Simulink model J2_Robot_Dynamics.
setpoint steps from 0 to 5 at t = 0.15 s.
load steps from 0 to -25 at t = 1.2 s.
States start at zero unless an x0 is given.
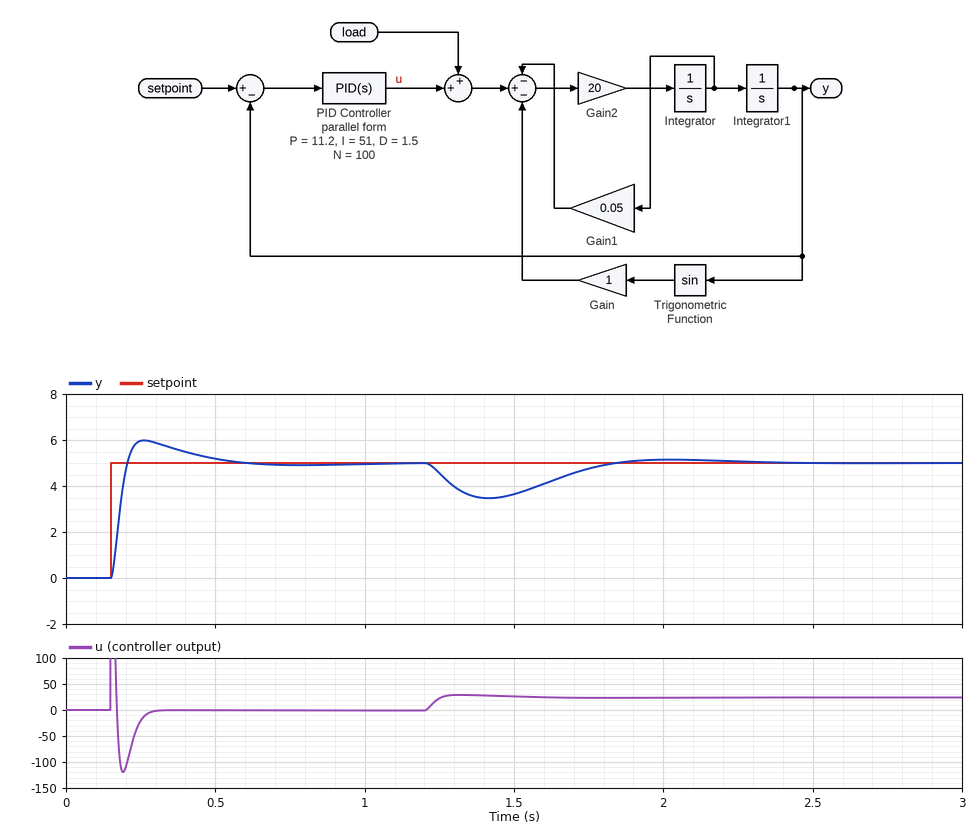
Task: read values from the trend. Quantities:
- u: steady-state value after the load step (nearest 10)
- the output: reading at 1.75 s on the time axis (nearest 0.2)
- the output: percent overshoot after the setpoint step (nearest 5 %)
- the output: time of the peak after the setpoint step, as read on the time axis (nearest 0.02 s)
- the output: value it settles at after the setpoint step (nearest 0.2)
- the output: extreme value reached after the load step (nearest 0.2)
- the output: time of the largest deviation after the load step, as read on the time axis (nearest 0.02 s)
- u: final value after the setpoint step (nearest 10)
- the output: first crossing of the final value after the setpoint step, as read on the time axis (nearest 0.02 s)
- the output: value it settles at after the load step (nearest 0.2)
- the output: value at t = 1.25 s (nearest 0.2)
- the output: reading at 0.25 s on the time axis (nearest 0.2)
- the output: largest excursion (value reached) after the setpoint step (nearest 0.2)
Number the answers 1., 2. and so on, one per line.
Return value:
1. 20
2. 4.8
3. 20 %
4. 0.26 s
5. 5.0
6. 3.4
7. 1.42 s
8. 0
9. 0.20 s
10. 5.0
11. 4.6
12. 6.0
13. 6.0
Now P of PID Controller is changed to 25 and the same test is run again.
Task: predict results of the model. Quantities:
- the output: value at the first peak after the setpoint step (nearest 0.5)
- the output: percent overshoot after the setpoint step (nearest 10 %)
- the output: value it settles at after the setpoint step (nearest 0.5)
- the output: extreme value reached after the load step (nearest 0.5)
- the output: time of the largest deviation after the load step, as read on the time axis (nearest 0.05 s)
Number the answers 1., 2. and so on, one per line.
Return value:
1. 6.5
2. 30 %
3. 5.0
4. 4.0
5. 1.35 s
